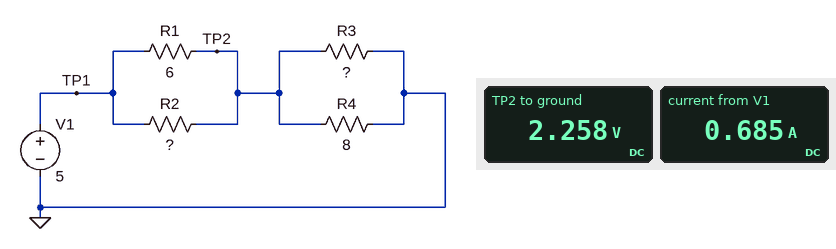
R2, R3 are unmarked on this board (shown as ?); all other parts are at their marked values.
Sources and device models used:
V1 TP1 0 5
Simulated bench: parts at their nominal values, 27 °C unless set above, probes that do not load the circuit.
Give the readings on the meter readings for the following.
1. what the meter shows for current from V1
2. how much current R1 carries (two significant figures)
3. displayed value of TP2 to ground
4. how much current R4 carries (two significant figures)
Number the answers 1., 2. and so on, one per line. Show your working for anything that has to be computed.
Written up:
1. 0.685 A
2. (5 V - 2.258 V) / 6 Ω = 460 mA
3. 2.258 V
4. (2.258 V) / 8 Ω = 280 mA
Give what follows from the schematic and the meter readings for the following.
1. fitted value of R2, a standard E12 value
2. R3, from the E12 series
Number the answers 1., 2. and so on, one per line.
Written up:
1. 12 Ω
2. 5.6 Ω
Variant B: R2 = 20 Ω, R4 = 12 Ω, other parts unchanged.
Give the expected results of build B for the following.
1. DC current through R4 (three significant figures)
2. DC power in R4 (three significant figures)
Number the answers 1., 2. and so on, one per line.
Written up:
1. 189 mA
2. 427 mW
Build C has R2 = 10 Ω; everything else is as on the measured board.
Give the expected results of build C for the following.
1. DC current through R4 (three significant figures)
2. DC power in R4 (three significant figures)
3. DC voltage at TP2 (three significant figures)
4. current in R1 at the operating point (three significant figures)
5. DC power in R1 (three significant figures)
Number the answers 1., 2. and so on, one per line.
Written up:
1. 292 mA
2. 683 mW
3. 2.34 V
4. 444 mA
5. 1.18 W
